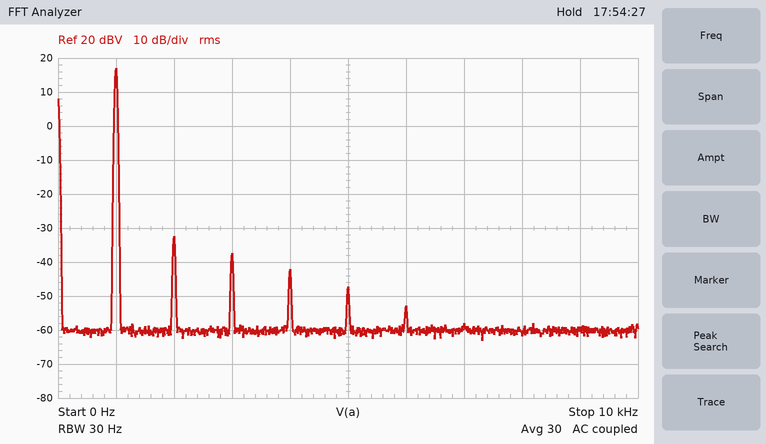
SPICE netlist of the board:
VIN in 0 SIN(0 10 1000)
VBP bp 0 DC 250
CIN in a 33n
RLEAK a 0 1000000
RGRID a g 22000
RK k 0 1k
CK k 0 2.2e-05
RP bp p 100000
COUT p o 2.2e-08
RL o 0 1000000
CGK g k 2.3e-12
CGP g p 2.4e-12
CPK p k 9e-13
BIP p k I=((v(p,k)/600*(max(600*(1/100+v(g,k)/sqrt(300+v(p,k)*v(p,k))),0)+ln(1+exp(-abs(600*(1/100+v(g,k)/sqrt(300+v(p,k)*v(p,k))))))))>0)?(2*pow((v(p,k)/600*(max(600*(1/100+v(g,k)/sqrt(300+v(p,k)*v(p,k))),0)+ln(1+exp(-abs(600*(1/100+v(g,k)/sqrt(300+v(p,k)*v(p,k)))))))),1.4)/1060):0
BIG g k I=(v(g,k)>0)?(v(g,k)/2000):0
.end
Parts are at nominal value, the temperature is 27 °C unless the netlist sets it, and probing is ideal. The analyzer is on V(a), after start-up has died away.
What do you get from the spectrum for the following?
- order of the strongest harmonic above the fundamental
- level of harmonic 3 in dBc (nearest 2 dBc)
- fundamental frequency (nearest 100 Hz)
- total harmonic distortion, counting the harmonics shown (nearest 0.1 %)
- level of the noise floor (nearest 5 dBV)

2
-54 dBc
1.0 kHz
0.4 %
-60 dBV
